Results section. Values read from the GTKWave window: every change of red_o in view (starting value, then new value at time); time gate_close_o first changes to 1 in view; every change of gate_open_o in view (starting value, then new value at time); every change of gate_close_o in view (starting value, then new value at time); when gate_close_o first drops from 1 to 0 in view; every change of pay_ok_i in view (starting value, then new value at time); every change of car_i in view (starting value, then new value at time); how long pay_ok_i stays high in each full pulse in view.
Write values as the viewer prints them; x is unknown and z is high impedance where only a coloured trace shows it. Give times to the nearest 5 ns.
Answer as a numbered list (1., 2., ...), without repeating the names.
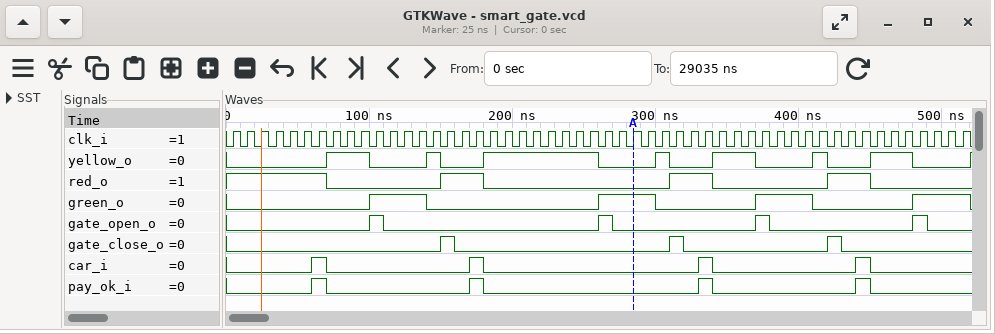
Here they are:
1. 1, 0 at 70 ns, 1 at 150 ns, 0 at 180 ns, 1 at 310 ns, 0 at 340 ns, 1 at 420 ns, 0 at 450 ns
2. 150 ns
3. 0, 1 at 100 ns, 0 at 110 ns, 1 at 260 ns, 0 at 270 ns, 1 at 370 ns, 0 at 380 ns, 1 at 480 ns, 0 at 490 ns
4. 0, 1 at 150 ns, 0 at 160 ns, 1 at 310 ns, 0 at 320 ns, 1 at 420 ns, 0 at 430 ns
5. 160 ns
6. 0, 1 at 60 ns, 0 at 70 ns, 1 at 170 ns, 0 at 180 ns, 1 at 330 ns, 0 at 340 ns, 1 at 440 ns, 0 at 450 ns
7. 0, 1 at 60 ns, 0 at 70 ns, 1 at 170 ns, 0 at 180 ns, 1 at 330 ns, 0 at 340 ns, 1 at 440 ns, 0 at 450 ns
8. 10 ns, 10 ns, 10 ns, 10 ns
